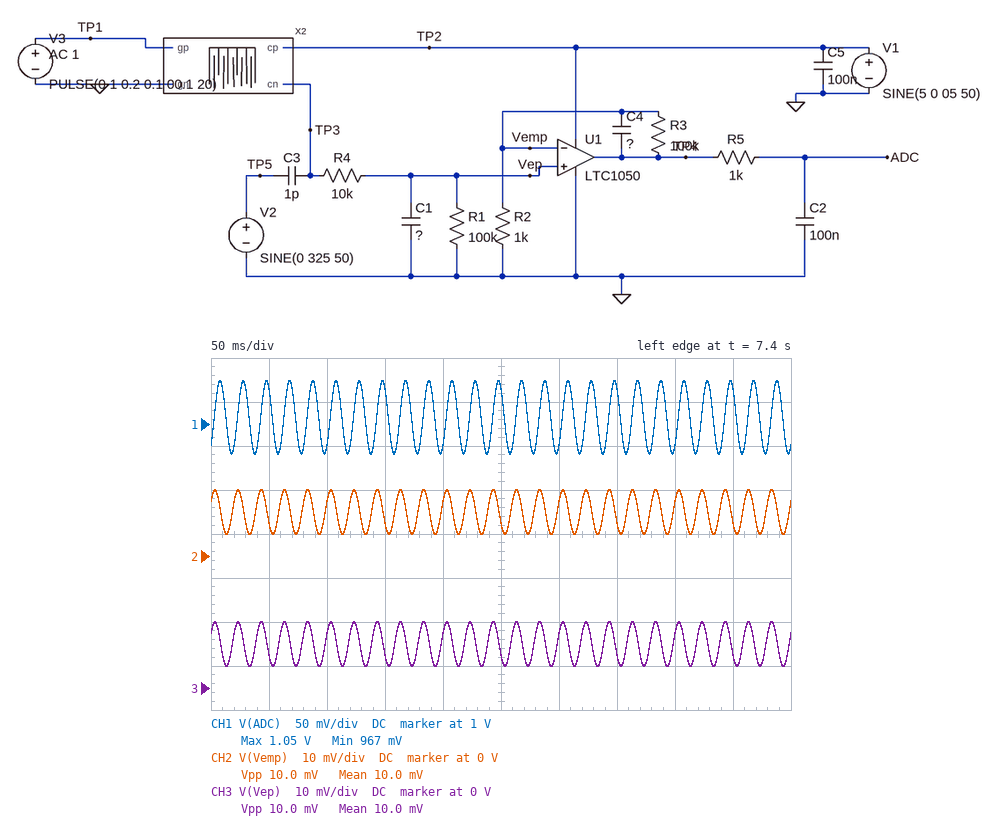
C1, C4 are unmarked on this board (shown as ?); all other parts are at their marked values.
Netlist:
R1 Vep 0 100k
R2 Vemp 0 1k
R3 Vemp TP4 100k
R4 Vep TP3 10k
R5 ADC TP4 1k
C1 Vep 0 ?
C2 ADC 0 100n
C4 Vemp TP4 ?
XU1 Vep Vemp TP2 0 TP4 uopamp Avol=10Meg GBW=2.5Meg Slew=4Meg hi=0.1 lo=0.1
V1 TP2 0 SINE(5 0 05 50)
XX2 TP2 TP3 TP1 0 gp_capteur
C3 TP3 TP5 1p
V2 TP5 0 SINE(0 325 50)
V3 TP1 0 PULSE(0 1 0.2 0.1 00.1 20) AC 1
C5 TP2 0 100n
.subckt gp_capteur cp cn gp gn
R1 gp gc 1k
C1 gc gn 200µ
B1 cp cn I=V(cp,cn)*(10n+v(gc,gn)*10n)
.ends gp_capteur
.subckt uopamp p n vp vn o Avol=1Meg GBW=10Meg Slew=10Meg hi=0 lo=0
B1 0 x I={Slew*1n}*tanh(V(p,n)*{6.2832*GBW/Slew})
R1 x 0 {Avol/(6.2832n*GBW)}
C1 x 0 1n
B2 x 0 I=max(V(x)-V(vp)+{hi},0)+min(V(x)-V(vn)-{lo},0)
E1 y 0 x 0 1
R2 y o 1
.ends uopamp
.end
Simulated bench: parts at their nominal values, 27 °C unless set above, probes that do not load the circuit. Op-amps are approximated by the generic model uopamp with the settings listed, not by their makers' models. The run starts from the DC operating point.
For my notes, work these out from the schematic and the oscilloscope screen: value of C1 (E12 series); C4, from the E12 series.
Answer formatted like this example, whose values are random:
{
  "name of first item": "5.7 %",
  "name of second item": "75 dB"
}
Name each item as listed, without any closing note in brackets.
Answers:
{
  "value of C1": "56 nF",
  "C4, from the E12 series": "390 nF"
}
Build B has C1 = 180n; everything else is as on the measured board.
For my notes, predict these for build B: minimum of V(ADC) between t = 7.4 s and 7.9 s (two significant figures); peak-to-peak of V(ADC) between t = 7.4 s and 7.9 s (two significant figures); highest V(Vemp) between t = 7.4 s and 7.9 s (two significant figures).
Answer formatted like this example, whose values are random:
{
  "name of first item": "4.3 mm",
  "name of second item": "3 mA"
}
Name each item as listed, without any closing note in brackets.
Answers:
{
  "minimum of V(ADC) between t = 7.4 s and 7.9 s": "990 mV",
  "peak-to-peak of V(ADC) between t = 7.4 s and 7.9 s": "29 mV",
  "highest V(Vemp) between t = 7.4 s and 7.9 s": "12 mV"
}
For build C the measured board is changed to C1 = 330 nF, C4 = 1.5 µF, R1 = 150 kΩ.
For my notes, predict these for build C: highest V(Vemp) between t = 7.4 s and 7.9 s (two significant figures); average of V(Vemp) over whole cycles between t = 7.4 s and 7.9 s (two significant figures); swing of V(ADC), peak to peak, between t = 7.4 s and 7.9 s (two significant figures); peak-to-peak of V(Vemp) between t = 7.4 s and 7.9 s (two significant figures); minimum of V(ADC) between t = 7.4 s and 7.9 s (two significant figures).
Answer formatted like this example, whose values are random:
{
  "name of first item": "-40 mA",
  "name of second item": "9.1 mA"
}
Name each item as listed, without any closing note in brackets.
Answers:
{
  "highest V(Vemp) between t = 7.4 s and 7.9 s": "16 mV",
  "average of V(Vemp) over whole cycles between t = 7.4 s and 7.9 s": "15 mV",
  "swing of V(ADC), peak to peak, between t = 7.4 s and 7.9 s": "4.6 mV",
  "peak-to-peak of V(Vemp) between t = 7.4 s and 7.9 s": "2.0 mV",
  "minimum of V(ADC) between t = 7.4 s and 7.9 s": "1.5 V"
}
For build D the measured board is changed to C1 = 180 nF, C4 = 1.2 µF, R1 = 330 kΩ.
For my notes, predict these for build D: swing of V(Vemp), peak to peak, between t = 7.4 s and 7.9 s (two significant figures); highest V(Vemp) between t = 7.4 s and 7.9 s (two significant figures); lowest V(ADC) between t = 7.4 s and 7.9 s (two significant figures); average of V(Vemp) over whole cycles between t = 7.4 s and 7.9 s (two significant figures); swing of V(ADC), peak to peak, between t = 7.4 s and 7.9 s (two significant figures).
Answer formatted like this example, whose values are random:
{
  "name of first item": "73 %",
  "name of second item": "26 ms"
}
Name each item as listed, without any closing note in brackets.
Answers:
{
  "swing of V(Vemp), peak to peak, between t = 7.4 s and 7.9 s": "3.6 mV",
  "highest V(Vemp) between t = 7.4 s and 7.9 s": "35 mV",
  "lowest V(ADC) between t = 7.4 s and 7.9 s": "3.3 V",
  "average of V(Vemp) over whole cycles between t = 7.4 s and 7.9 s": "33 mV",
  "swing of V(ADC), peak to peak, between t = 7.4 s and 7.9 s": "10 mV"
}
